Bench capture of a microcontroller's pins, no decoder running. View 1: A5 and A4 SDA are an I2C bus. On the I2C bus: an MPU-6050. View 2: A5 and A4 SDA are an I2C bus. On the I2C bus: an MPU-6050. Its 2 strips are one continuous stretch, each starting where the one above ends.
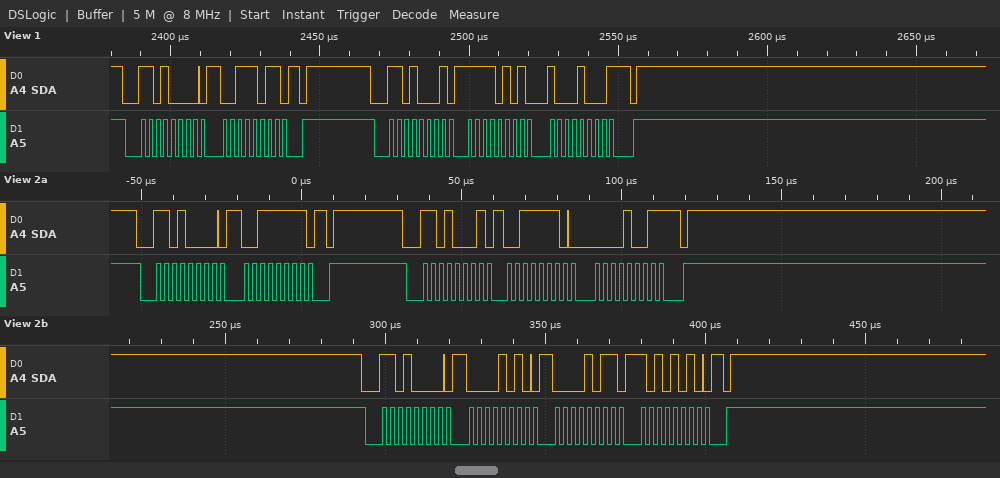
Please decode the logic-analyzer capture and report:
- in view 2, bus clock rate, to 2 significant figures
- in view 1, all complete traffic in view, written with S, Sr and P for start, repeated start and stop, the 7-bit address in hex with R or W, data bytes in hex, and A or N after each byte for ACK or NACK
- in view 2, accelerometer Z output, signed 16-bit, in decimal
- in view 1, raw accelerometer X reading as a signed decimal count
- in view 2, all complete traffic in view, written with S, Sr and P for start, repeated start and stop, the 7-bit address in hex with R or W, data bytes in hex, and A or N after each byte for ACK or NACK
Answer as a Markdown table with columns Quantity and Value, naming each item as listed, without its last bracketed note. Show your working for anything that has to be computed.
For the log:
| Quantity | Value |
|---|---|
| in view 2, bus clock rate, to 2 significant figures | 400 kHz |
| in view 1, all complete traffic in view, written with S, Sr and P for start, repeated start and stop, the 7-bit address in hex with R or W, data bytes in hex, and A or N after each byte for ACK or NACK | S 68W A 3B A P S 68R A F5 A 88 N P |
| in view 2, accelerometer Z output, signed 16-bit, in decimal | 0x3E09 = 15881 |
| in view 1, raw accelerometer X reading as a signed decimal count | 0xF588 = -2680 |
| in view 2, all complete traffic in view, written with S, Sr and P for start, repeated start and stop, the 7-bit address in hex with R or W, data bytes in hex, and A or N after each byte for ACK or NACK | S 68W A 3F A P S 68R A 3E A 09 N P S 68W A 0A A 0B A AA A P |
